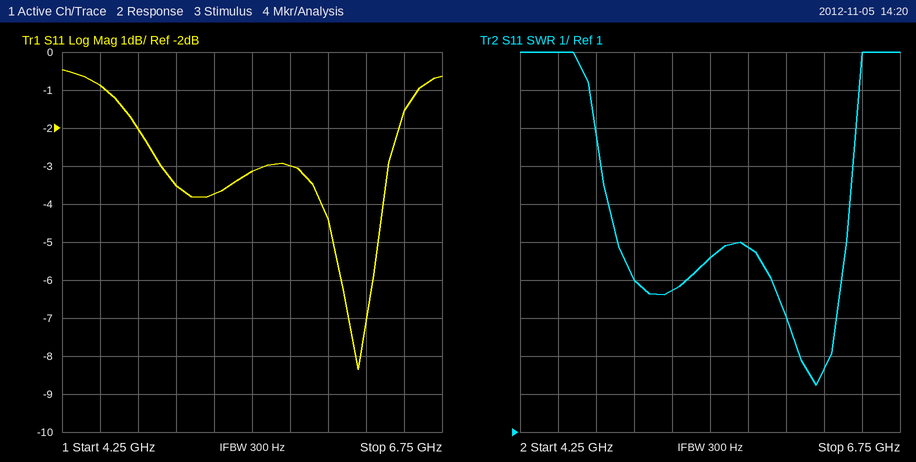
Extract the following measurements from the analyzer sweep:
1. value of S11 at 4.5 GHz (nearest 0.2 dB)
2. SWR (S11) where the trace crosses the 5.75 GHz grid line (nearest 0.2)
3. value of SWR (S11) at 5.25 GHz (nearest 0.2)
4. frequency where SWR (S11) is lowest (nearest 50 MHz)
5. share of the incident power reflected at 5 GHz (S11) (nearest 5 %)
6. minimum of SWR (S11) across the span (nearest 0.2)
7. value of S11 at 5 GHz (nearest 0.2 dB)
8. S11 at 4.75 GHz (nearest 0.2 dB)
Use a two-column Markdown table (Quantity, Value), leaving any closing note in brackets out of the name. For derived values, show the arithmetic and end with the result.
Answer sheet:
| Quantity | Value |
|---|---|
| value of S11 at 4.5 GHz | -0.8 dB |
| SWR (S11) where the trace crosses the 5.75 GHz grid line | 5.8 |
| value of SWR (S11) at 5.25 GHz | 4.8 |
| frequency where SWR (S11) is lowest | 6.20 GHz |
| share of the incident power reflected at 5 GHz (S11) | 10^(-3.6/10) ≈ 43.7 %, so 45 % to the nearest 5 % |
| minimum of SWR (S11) across the span | 2.2 |
| value of S11 at 5 GHz | -3.6 dB |
| S11 at 4.75 GHz | -2.0 dB |
